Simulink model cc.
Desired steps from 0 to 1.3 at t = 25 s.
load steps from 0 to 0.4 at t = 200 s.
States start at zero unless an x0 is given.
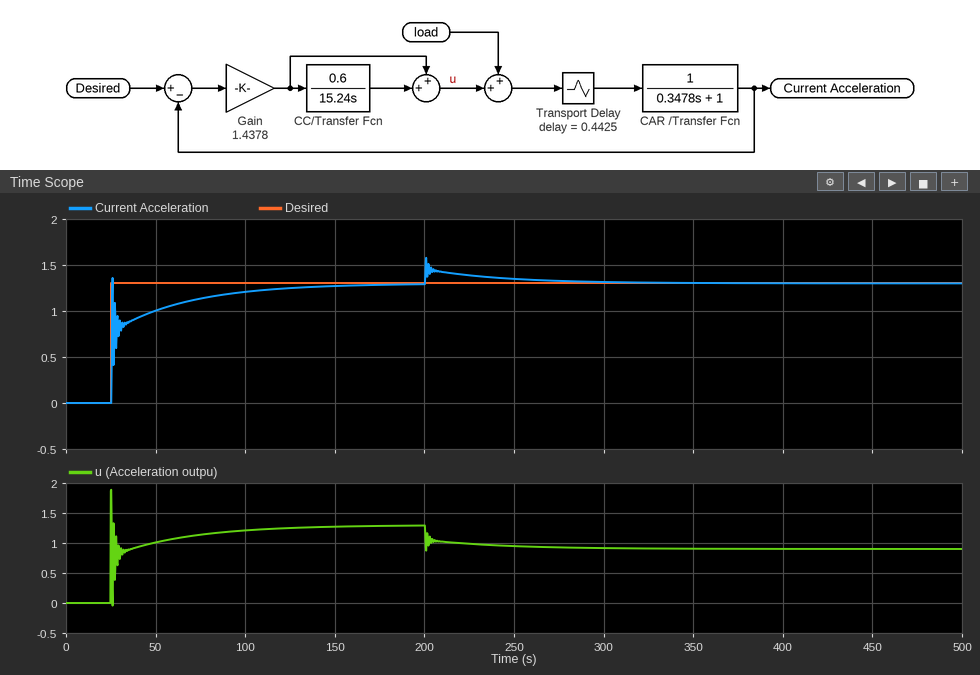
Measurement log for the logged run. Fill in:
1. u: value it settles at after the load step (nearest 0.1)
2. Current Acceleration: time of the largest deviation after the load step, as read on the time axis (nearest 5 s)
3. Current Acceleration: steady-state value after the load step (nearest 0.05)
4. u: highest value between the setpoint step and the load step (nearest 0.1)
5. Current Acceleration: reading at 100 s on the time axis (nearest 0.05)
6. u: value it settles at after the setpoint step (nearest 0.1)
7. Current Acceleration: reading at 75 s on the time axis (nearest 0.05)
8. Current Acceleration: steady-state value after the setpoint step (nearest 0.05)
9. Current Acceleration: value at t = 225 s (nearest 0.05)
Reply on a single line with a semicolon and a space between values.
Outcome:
0.9; 200 s; 1.30; 1.9; 1.20; 1.3; 1.15; 1.30; 1.40
